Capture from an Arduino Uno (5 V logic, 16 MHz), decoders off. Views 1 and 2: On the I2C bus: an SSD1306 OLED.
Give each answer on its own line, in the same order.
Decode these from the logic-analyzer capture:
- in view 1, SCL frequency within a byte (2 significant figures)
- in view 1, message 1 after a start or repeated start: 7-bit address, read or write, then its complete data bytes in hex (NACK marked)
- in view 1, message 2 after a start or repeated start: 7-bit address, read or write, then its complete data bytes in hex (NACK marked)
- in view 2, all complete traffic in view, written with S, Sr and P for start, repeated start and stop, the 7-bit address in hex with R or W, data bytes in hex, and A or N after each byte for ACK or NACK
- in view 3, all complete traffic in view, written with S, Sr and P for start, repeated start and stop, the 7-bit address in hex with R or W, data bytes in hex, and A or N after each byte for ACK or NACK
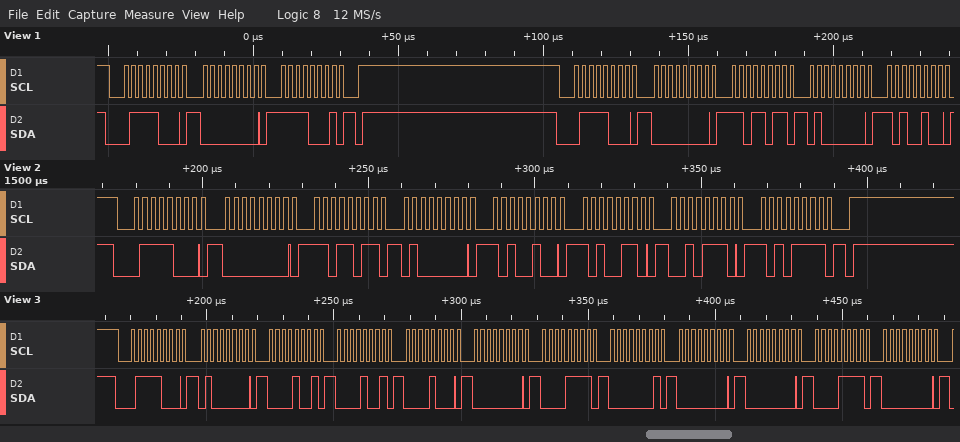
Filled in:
400 kHz
0x3C write: 00 F1
0x3C write: 00 DB 40 A4
S 3CW A 00 A DB A 40 A A4 A A6 A 2E A AF A P
S 3CW A 40 A 09 A 09 A 08 A 00 A 0F A 01 A 00 A 00 A 0F A 00 A
